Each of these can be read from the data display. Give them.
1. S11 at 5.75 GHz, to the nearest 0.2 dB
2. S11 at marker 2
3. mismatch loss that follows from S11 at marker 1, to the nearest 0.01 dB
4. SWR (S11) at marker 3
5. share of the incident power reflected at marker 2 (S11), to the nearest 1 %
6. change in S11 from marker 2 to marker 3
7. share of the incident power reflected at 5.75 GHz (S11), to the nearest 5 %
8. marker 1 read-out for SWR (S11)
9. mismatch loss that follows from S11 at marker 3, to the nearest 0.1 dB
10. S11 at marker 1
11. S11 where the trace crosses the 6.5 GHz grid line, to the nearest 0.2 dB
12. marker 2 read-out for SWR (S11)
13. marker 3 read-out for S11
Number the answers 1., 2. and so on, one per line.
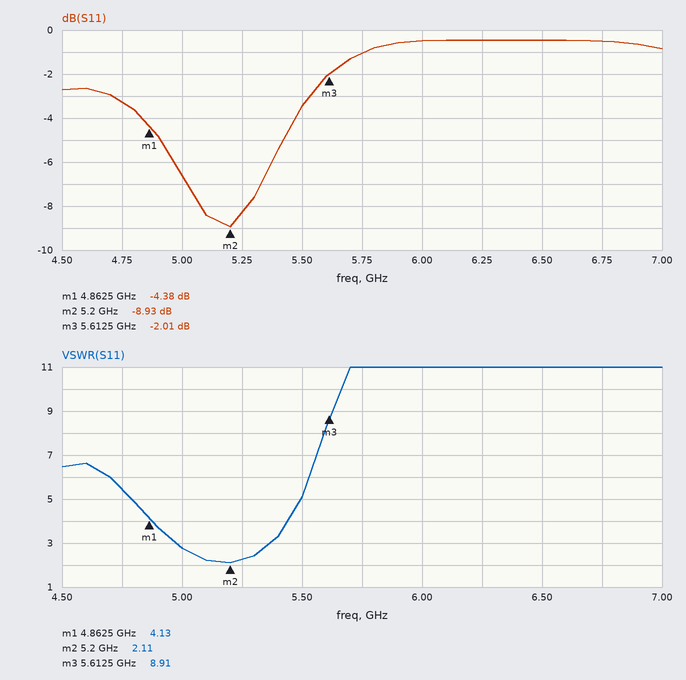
1. -1.0 dB
2. -8.93 dB
3. 1.97 dB
4. 8.91
5. 13 %
6. 6.92 dB
7. 80 %
8. 4.13
9. 4.3 dB
10. -4.38 dB
11. -0.4 dB
12. 2.11
13. -2.01 dB
